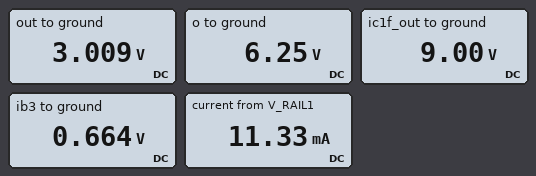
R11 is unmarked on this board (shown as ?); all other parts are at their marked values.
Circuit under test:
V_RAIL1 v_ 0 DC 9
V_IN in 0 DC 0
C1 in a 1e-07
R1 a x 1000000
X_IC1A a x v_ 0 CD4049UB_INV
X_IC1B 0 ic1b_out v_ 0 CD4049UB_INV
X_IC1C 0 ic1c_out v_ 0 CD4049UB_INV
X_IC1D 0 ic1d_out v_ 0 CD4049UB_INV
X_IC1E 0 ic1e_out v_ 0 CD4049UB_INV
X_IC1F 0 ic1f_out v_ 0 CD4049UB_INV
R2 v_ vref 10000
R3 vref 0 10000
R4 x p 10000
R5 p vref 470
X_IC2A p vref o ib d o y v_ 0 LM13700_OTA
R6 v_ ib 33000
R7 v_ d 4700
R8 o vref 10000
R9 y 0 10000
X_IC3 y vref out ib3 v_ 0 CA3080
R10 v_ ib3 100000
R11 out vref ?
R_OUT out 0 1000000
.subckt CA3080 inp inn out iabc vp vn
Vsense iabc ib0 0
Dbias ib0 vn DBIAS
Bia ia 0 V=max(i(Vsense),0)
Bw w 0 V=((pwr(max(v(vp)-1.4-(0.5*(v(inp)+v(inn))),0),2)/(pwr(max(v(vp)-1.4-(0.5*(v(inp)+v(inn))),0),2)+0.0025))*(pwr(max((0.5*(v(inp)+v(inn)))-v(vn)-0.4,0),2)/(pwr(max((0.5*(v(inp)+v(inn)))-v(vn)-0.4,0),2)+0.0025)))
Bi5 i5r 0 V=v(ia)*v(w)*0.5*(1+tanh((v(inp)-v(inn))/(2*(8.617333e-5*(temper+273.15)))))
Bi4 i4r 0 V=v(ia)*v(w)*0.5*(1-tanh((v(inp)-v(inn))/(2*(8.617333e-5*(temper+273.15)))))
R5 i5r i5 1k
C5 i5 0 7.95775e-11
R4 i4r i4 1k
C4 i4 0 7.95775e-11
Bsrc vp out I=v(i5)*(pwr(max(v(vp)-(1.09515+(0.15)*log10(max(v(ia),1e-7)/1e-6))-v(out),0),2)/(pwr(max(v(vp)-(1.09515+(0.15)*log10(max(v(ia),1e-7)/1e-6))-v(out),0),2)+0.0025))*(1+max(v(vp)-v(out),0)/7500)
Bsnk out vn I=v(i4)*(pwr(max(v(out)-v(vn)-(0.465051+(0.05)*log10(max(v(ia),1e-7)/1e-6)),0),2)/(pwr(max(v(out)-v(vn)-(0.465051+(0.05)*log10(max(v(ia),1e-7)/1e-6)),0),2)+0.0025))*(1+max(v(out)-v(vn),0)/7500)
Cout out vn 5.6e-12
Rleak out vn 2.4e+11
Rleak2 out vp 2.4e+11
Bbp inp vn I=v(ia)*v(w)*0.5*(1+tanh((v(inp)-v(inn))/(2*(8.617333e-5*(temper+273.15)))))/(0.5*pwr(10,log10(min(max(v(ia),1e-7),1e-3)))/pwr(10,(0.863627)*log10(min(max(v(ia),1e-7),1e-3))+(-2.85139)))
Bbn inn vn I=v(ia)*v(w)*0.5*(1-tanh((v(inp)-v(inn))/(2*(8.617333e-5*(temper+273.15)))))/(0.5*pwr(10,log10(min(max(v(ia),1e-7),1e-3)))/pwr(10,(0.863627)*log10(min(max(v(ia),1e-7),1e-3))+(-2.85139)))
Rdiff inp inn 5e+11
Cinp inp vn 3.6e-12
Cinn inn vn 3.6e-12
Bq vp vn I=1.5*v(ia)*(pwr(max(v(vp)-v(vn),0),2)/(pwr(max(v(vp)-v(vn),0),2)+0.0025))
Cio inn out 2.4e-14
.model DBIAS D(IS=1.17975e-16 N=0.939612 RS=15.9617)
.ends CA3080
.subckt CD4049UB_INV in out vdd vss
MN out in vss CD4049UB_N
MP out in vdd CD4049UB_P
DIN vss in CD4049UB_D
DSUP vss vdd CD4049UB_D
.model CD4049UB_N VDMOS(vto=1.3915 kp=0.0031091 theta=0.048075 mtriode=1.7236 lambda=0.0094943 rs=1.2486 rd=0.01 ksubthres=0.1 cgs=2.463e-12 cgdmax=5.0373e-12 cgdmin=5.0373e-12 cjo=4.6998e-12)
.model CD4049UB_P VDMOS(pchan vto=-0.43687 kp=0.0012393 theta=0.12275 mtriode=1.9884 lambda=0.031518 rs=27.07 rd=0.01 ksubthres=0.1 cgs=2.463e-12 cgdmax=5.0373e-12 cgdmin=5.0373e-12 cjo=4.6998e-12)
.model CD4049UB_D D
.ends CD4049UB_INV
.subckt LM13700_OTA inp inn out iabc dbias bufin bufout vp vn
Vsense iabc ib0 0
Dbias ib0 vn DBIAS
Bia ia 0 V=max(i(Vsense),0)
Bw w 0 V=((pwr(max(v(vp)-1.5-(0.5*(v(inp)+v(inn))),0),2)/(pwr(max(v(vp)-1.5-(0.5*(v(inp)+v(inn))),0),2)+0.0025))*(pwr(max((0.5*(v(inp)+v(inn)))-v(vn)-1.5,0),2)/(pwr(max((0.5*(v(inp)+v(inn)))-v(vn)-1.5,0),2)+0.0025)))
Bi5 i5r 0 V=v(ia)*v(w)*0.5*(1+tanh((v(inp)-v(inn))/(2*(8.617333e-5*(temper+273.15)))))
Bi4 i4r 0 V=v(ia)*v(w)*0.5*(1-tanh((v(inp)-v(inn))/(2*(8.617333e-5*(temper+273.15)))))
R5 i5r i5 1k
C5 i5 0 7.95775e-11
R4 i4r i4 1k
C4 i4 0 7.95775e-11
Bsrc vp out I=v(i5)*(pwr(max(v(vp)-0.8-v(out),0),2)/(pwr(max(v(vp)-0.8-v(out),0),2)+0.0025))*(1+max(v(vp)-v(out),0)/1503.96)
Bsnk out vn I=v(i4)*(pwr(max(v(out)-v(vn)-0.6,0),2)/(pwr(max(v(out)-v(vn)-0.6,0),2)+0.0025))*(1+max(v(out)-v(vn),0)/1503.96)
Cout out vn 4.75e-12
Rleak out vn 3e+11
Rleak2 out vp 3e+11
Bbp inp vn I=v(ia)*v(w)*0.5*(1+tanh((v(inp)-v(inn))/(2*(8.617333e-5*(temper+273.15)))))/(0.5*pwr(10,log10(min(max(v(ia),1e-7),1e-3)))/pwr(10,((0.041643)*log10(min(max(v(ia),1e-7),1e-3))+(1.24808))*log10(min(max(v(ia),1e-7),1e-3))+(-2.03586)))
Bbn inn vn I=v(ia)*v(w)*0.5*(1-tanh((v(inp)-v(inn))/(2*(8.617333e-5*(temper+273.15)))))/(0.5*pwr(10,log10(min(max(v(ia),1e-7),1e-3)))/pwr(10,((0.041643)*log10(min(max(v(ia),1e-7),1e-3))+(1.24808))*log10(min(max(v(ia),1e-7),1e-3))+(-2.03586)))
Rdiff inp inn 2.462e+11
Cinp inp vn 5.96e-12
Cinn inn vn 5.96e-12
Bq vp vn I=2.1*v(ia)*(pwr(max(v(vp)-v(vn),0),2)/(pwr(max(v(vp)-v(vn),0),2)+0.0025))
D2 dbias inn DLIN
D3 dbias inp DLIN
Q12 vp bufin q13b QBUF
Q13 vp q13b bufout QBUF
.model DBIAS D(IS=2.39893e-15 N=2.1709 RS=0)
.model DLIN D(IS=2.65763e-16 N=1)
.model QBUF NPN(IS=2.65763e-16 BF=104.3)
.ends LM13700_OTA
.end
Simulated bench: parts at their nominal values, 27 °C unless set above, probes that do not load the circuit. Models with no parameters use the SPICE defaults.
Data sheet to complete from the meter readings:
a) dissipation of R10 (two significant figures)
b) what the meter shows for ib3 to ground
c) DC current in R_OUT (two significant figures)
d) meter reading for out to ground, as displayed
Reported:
690 µW
0.664 V
3.0 µA
3.009 V
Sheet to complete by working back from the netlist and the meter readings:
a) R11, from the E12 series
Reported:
33 kΩ
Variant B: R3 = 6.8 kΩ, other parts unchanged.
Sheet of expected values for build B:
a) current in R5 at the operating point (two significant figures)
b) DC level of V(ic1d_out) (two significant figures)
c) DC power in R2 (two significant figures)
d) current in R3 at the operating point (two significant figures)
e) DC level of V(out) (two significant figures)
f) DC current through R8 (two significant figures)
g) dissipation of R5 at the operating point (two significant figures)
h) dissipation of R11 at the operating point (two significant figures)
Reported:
41 µA
9.0 V
1.3 mW
800 µA
2.6 V
81 µA
780 nW
240 µW
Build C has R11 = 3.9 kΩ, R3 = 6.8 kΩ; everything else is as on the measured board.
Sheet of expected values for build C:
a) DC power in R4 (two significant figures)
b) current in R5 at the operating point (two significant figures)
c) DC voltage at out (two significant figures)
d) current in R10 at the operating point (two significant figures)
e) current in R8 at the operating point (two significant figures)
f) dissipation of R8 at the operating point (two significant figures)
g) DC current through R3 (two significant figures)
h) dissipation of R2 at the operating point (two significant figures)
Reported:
230 µW
41 µA
5.1 V
83 µA
81 µA
66 µW
800 µA
1.3 mW
